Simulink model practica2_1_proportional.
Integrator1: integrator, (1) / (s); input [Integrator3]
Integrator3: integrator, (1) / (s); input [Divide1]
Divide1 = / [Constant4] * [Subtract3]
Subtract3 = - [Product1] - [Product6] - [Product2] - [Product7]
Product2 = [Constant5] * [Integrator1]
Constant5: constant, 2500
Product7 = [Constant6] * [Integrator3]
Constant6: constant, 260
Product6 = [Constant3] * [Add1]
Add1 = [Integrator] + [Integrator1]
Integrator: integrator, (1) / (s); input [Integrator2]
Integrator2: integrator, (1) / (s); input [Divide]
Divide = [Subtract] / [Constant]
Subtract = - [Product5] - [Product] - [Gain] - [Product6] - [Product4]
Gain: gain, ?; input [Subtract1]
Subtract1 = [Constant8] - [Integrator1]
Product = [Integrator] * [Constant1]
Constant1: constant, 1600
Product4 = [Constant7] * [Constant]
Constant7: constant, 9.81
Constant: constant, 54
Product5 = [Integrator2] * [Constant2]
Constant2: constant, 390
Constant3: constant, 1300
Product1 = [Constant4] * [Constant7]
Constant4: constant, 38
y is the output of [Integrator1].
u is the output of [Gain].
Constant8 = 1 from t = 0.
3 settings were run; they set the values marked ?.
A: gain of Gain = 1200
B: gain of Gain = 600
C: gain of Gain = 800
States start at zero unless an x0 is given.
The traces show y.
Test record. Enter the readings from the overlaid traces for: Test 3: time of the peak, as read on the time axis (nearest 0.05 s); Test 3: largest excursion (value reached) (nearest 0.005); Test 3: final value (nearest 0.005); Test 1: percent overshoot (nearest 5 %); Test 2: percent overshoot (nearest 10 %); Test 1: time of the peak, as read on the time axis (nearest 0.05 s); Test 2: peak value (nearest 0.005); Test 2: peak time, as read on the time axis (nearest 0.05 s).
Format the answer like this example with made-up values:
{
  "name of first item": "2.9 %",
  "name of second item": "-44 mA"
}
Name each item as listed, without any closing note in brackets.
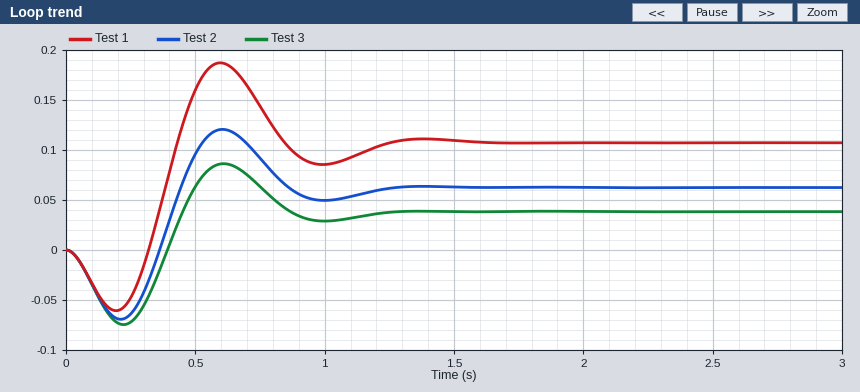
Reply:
{
  "Test 3: time of the peak, as read on the time axis": "0.60 s",
  "Test 3: largest excursion (value reached)": "0.085",
  "Test 3: final value": "0.040",
  "Test 1: percent overshoot": "75 %",
  "Test 2: percent overshoot": "90 %",
  "Test 1: time of the peak, as read on the time axis": "0.60 s",
  "Test 2: peak value": "0.120",
  "Test 2: peak time, as read on the time axis": "0.60 s"
}
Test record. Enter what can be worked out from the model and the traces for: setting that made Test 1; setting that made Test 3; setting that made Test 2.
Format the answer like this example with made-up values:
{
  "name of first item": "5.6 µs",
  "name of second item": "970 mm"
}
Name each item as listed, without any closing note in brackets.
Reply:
{
  "setting that made Test 1": "A",
  "setting that made Test 3": "B",
  "setting that made Test 2": "C"
}
